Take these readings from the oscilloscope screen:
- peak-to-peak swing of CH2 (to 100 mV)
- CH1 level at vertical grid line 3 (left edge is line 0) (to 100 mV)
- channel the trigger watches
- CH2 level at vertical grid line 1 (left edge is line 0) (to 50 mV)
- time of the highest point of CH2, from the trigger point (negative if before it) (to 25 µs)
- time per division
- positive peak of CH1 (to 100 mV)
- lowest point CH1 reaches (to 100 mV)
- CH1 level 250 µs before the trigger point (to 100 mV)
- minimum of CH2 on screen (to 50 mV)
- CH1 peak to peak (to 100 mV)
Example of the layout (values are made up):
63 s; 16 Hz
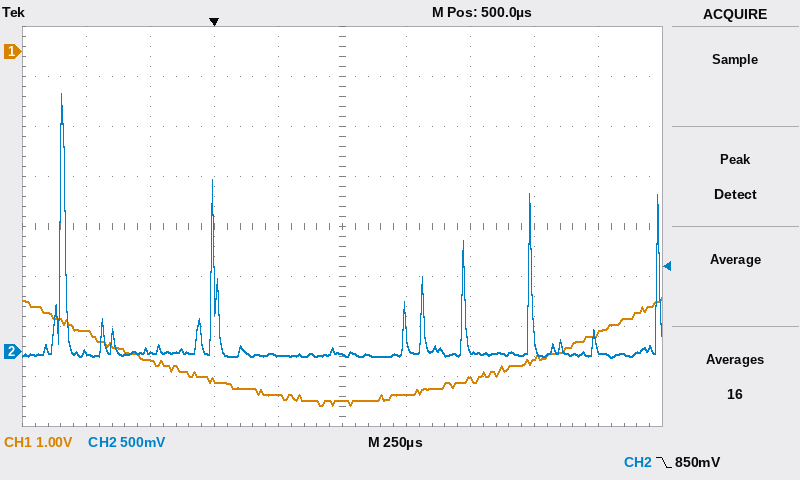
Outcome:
2.60 V; -6.6 V; CH2; 0 mV; -600 µs; 250 µs; -4.9 V; -7.1 V; -6.2 V; -50 mV; 2.2 V
